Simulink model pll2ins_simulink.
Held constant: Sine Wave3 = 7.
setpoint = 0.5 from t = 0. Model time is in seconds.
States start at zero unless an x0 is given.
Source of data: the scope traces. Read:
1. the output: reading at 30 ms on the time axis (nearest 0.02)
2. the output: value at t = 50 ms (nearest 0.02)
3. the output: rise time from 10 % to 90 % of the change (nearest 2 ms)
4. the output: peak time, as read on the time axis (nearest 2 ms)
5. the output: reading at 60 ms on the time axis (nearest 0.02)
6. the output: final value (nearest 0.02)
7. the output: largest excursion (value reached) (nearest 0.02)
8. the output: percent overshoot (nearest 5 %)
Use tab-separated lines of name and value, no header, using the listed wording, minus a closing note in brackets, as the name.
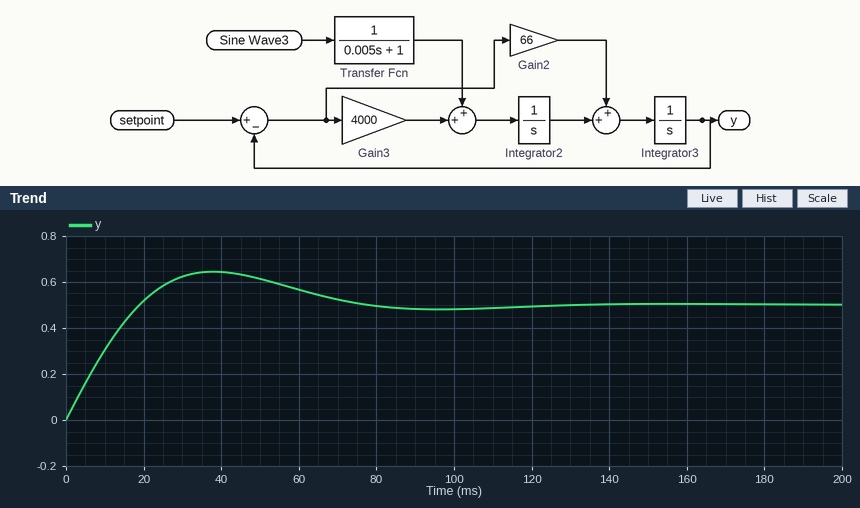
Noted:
the output: reading at 30 ms on the time axis	0.62
the output: value at t = 50 ms	0.62
the output: rise time from 10 % to 90 % of the change	14 ms
the output: peak time, as read on the time axis	38 ms
the output: reading at 60 ms on the time axis	0.56
the output: final value	0.50
the output: largest excursion (value reached)	0.64
the output: percent overshoot	30 %
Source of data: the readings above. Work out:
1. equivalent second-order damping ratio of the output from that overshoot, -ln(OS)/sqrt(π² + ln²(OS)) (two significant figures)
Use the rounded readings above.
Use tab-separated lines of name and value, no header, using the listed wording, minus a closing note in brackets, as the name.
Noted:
equivalent second-order damping ratio of the output from that overshoot, -ln(OS)/sqrt(π² + ln²(OS))	0.36
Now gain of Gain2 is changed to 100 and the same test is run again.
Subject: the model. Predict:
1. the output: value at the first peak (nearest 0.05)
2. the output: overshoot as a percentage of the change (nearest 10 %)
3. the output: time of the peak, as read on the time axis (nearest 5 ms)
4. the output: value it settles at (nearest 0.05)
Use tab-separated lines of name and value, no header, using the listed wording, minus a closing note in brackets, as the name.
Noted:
the output: value at the first peak	0.60
the output: overshoot as a percentage of the change	20 %
the output: time of the peak, as read on the time axis	35 ms
the output: value it settles at	0.50
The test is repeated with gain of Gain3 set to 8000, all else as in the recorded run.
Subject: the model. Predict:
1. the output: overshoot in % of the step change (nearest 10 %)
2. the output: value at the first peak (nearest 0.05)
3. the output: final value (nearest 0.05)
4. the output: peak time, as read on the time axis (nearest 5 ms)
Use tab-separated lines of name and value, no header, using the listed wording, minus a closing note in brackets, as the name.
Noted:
the output: overshoot in % of the step change	40 %
the output: value at the first peak	0.70
the output: final value	0.50
the output: peak time, as read on the time axis	30 ms
